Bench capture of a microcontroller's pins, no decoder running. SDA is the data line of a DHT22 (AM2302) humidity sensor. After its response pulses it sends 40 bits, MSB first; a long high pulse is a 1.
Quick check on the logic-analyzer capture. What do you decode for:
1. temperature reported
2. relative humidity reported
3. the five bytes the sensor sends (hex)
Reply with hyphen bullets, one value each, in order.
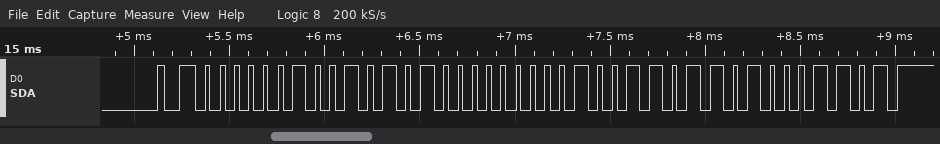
- 31.0 °C
- 59.6 %
- 02 54 01 36 8D
